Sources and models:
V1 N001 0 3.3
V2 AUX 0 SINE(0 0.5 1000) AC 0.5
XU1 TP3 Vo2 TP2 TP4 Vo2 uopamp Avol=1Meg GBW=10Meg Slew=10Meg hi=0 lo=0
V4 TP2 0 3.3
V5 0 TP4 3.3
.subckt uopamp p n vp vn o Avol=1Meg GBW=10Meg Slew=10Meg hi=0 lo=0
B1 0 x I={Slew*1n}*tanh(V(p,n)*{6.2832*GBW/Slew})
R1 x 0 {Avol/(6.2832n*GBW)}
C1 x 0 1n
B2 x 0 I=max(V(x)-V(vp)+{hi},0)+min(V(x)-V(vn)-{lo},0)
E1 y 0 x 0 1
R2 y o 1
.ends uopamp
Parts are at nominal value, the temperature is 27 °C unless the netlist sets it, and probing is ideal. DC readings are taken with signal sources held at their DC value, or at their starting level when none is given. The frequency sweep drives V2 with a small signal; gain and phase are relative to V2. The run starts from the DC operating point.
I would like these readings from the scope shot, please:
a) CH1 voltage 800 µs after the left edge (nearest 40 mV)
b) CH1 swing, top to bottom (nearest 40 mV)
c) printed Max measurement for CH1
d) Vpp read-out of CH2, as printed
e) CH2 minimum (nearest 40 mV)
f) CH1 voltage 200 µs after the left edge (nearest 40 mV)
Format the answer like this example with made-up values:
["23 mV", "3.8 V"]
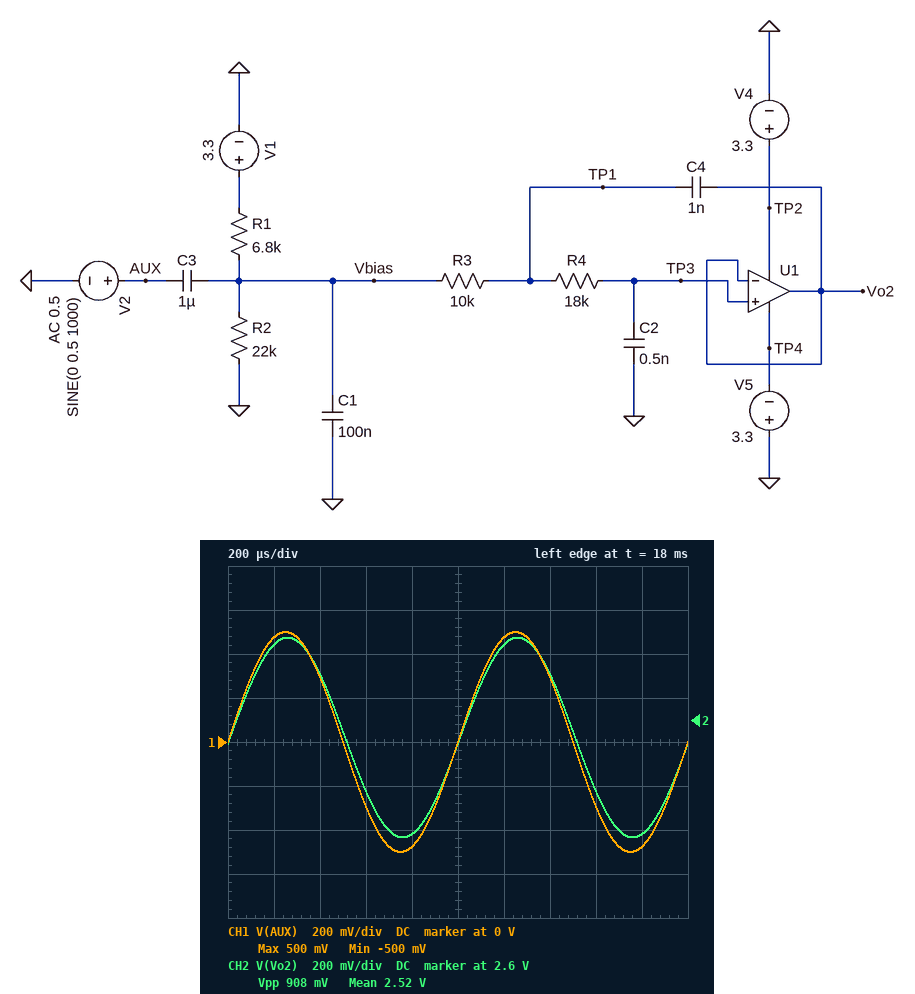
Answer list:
["-480 mV", "1.00 V", "500 mV", "908 mV", "2.08 V", "480 mV"]
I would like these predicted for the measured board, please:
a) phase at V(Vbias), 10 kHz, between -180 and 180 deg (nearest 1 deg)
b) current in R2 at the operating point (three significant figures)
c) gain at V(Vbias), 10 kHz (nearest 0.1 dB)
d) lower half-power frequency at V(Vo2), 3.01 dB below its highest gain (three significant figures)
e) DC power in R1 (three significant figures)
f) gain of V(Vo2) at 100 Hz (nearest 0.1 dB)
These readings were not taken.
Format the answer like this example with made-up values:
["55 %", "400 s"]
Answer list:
["0 deg", "115 µA", "-0.8 dB", "27.8 Hz", "89.3 µW", "-1.2 dB"]
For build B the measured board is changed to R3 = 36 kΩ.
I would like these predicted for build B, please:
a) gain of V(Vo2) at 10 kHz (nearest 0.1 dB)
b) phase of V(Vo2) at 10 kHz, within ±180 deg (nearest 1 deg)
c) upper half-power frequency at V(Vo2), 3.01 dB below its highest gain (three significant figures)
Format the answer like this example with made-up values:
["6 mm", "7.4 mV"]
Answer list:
["-5.5 dB", "-99 deg", "8.32 kHz"]
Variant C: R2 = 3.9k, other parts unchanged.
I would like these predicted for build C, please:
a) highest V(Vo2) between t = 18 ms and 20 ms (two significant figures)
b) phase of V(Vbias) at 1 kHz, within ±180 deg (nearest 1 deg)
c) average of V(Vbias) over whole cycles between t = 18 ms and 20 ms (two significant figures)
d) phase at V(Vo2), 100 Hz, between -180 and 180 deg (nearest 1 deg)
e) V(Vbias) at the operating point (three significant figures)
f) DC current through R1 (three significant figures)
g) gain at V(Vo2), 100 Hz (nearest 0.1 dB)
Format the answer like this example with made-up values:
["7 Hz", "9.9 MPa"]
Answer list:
["1.7 V", "3 deg", "1.2 V", "30 deg", "1.20 V", "308 µA", "-2.1 dB"]
